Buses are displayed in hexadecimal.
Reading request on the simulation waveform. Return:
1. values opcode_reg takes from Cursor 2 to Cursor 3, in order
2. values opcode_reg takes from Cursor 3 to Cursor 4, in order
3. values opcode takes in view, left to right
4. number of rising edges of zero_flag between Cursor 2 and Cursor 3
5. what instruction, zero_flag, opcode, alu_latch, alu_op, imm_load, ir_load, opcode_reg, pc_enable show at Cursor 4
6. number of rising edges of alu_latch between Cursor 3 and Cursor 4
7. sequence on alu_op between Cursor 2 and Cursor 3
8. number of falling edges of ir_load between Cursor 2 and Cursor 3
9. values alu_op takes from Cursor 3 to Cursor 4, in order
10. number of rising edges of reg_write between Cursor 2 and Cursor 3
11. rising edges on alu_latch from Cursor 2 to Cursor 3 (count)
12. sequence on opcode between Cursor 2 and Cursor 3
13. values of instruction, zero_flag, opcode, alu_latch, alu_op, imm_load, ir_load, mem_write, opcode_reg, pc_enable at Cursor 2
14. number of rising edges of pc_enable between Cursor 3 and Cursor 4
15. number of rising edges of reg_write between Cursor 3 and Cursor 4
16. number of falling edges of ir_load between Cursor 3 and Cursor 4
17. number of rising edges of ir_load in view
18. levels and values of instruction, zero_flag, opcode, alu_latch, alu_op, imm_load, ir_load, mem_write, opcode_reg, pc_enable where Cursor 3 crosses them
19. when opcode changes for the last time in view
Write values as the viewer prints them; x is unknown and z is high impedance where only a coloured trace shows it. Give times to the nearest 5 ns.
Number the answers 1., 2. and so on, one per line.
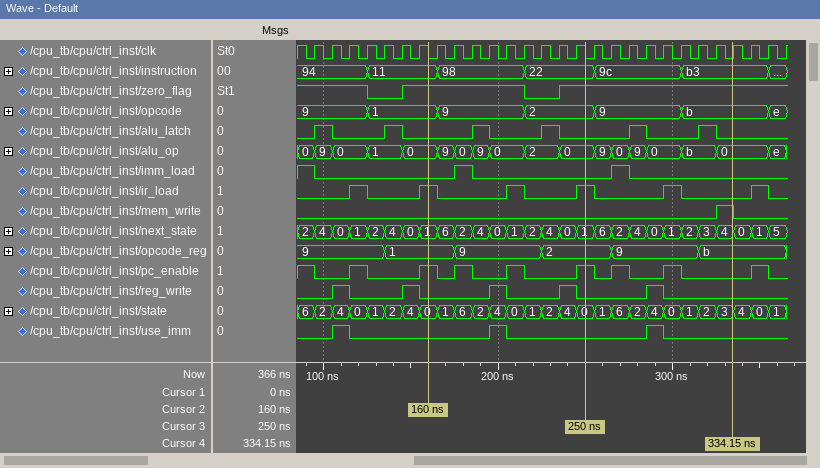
1. 1, 9, 2
2. 2, 9, b
3. 9, 1, 9, 2, 9, b, e
4. 1
5. instruction=b3, zero_flag=1, opcode=b, alu_latch=0, alu_op=0, imm_load=0, ir_load=0, opcode_reg=b, pc_enable=0
6. 2
7. 0, 9, 0, 9, 0, 2, 0
8. 2
9. 0, 9, 0, 9, 0, b, 0
10. 2
11. 2
12. 1, 9, 2
13. instruction=11, zero_flag=1, opcode=1, alu_latch=0, alu_op=0, imm_load=0, ir_load=1, mem_write=0, opcode_reg=1, pc_enable=1
14. 2
15. 1
16. 2
17. 6
18. instruction=22, zero_flag=1, opcode=2, alu_latch=0, alu_op=0, imm_load=0, ir_load=1, mem_write=0, opcode_reg=2, pc_enable=1
19. 355 ns
